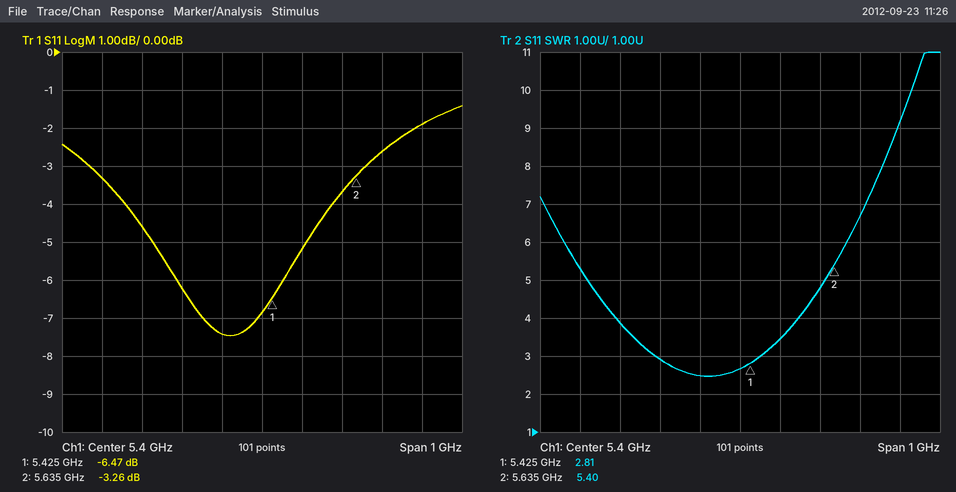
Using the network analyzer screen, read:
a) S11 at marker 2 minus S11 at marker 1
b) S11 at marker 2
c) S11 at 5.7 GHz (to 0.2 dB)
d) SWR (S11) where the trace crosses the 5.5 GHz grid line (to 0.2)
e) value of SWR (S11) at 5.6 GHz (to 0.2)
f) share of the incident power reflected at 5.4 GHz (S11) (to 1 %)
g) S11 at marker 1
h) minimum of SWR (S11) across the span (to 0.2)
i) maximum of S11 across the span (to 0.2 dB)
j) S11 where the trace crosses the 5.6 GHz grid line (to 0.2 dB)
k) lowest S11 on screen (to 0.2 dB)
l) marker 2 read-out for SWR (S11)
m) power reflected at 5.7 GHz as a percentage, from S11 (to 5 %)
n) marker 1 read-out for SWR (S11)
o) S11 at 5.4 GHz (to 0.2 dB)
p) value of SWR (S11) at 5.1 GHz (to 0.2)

3.21 dB
-3.26 dB
-2.6 dB
3.4
4.8
21 %
-6.47 dB
2.4
-1.4 dB
-3.6 dB
-7.4 dB
5.40
55 %
2.81
-6.8 dB
3.8
